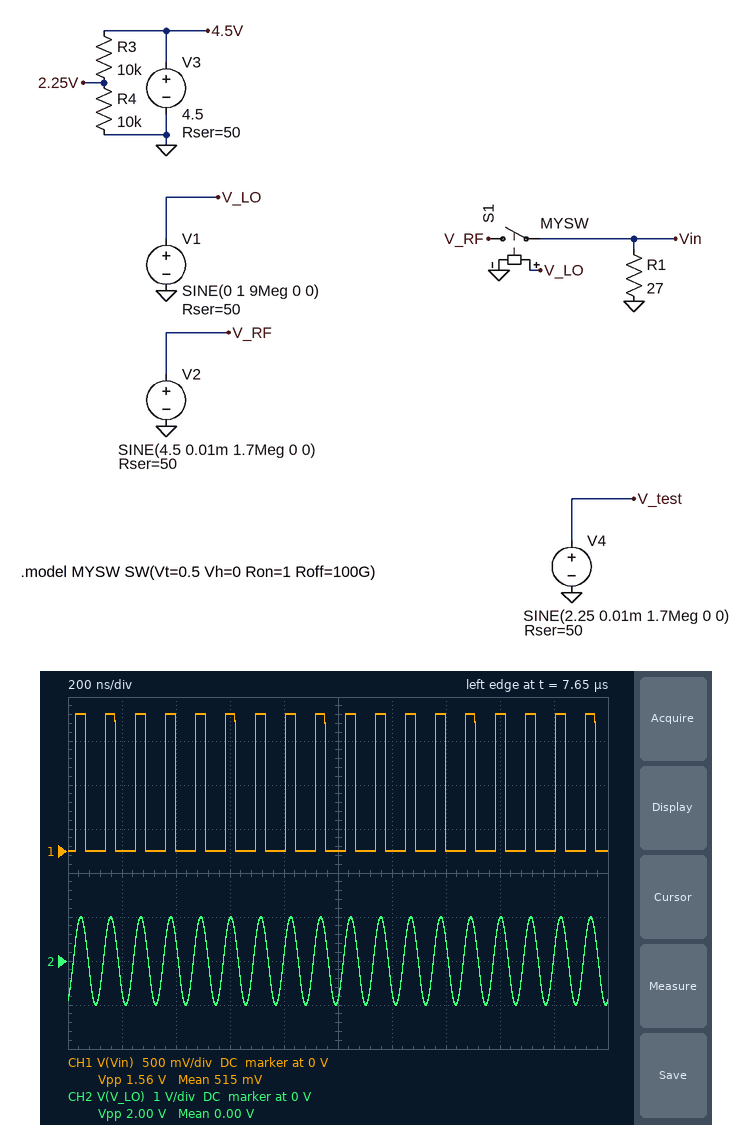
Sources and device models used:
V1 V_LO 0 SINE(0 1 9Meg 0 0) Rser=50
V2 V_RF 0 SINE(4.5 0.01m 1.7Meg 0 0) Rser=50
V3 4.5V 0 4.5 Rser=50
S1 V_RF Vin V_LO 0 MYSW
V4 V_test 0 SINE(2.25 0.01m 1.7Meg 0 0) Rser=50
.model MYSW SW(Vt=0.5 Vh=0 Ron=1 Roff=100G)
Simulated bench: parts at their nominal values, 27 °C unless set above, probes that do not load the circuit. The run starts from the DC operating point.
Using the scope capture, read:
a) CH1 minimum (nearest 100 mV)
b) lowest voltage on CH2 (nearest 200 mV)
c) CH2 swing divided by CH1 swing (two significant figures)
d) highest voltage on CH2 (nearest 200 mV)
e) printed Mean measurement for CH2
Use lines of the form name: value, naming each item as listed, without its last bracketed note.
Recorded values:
CH1 minimum: 0 V
lowest voltage on CH2: -1.0 V
CH2 swing divided by CH1 swing: 1.3
highest voltage on CH2: 1.0 V
printed Mean measurement for CH2: 0.00 V
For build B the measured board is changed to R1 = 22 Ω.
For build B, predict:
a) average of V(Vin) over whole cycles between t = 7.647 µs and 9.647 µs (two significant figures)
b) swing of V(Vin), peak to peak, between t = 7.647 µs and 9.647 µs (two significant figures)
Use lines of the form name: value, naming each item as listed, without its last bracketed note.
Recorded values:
average of V(Vin) over whole cycles between t = 7.647 µs and 9.647 µs: 450 mV
swing of V(Vin), peak to peak, between t = 7.647 µs and 9.647 µs: 1.4 V
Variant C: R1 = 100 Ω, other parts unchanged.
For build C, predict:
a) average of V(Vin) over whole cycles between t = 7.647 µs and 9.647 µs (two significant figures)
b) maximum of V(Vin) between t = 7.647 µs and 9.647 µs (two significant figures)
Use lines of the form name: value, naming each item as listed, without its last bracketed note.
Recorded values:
average of V(Vin) over whole cycles between t = 7.647 µs and 9.647 µs: 990 mV
maximum of V(Vin) between t = 7.647 µs and 9.647 µs: 3.0 V
